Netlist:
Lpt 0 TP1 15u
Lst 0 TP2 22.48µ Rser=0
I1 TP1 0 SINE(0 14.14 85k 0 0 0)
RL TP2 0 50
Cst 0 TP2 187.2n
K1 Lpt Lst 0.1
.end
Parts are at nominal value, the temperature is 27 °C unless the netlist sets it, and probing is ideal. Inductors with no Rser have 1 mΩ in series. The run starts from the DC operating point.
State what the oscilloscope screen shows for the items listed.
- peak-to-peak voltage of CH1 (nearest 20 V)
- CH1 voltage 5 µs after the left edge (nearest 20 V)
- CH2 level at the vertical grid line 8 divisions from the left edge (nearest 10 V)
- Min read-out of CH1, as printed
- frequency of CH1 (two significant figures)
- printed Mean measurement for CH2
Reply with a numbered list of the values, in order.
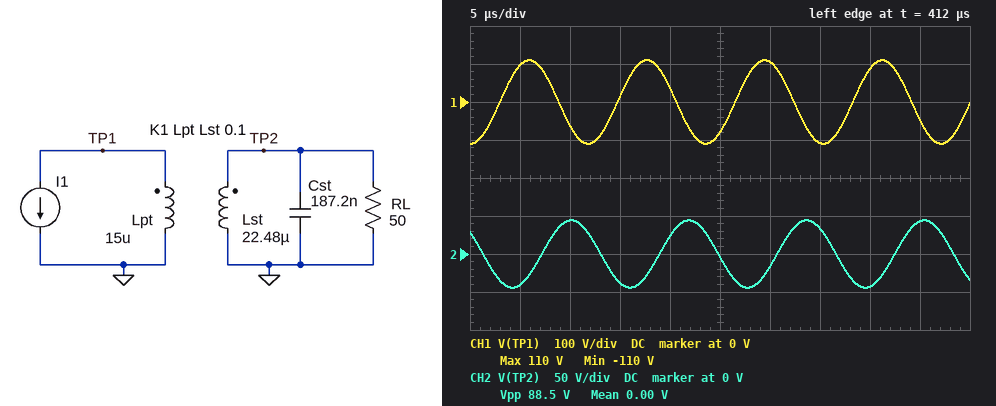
1. 220 V
2. 100 V
3. -40 V
4. -110 V
5. 85 kHz
6. 0.00 V
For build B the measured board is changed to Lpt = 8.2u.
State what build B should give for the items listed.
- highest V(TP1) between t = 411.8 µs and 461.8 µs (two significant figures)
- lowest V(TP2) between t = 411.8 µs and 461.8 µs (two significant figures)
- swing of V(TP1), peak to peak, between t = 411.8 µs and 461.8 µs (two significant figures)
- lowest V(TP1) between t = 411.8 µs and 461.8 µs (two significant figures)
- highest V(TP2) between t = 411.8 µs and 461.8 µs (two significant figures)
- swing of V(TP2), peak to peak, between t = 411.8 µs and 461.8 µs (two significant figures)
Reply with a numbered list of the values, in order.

1. 60 V
2. -33 V
3. 120 V
4. -60 V
5. 33 V
6. 66 V
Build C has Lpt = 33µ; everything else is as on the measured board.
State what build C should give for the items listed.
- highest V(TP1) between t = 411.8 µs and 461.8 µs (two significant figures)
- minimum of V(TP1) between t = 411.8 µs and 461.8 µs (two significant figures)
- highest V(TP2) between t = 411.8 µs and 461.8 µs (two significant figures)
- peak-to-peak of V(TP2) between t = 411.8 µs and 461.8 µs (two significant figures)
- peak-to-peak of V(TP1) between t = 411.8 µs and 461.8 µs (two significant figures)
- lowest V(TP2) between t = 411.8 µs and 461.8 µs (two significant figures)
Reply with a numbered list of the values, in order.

1. 240 V
2. -240 V
3. 66 V
4. 130 V
5. 480 V
6. -66 V
